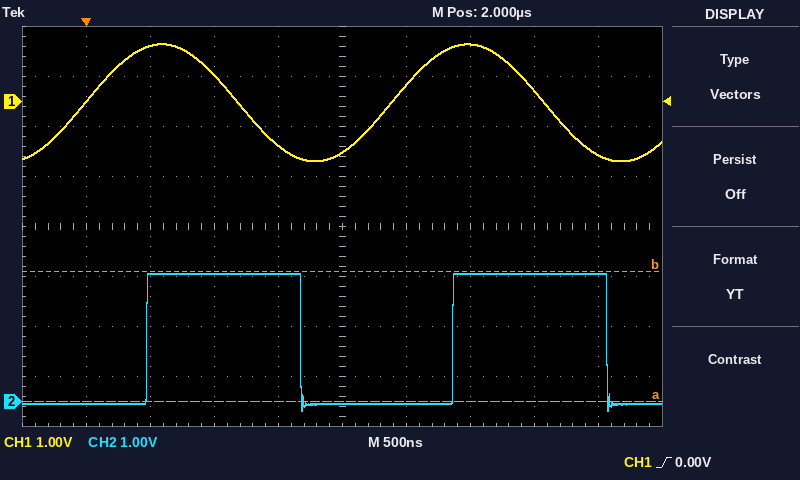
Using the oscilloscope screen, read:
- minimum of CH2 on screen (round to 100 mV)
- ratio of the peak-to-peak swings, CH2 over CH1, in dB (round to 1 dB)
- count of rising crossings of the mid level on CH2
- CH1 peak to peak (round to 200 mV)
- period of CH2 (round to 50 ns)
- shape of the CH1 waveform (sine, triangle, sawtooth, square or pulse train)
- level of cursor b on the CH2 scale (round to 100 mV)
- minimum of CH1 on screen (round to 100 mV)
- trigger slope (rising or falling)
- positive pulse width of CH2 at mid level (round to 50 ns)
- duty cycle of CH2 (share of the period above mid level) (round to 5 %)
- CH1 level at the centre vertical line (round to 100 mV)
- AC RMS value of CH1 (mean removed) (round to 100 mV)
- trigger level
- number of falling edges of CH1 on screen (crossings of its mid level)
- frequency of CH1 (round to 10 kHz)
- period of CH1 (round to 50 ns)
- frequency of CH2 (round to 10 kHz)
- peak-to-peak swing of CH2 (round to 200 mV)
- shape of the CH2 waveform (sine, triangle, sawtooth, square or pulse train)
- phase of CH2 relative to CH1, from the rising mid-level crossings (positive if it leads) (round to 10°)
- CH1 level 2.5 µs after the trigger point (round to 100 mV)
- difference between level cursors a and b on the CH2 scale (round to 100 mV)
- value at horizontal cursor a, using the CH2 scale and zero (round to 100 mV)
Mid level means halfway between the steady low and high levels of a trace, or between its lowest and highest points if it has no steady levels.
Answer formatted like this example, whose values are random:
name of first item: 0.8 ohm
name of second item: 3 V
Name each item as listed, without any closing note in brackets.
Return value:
minimum of CH2 on screen: -200 mV
ratio of the peak-to-peak swings, CH2 over CH1, in dB: 1 dB
count of rising crossings of the mid level on CH2: 2
CH1 peak to peak: 2.4 V
period of CH2: 2.40 µs
shape of the CH1 waveform: sine
level of cursor b on the CH2 scale: 2.6 V
minimum of CH1 on screen: -1.2 V
trigger slope: rising
positive pulse width of CH2 at mid level: 1.20 µs
duty cycle of CH2 (share of the period above mid level): 50 %
CH1 level at the centre vertical line: -1.0 V
AC RMS value of CH1 (mean removed): 800 mV
trigger level: 0.00 V
number of falling edges of CH1 on screen: 2
frequency of CH1: 420 kHz
period of CH1: 2.40 µs
frequency of CH2: 420 kHz
peak-to-peak swing of CH2: 2.8 V
shape of the CH2 waveform: square
phase of CH2 relative to CH1, from the rising mid-level crossings (positive if it leads): -70°
CH1 level 2.5 µs after the trigger point: 300 mV
difference between level cursors a and b on the CH2 scale: 2.6 V
value at horizontal cursor a, using the CH2 scale and zero: 0.0 V
